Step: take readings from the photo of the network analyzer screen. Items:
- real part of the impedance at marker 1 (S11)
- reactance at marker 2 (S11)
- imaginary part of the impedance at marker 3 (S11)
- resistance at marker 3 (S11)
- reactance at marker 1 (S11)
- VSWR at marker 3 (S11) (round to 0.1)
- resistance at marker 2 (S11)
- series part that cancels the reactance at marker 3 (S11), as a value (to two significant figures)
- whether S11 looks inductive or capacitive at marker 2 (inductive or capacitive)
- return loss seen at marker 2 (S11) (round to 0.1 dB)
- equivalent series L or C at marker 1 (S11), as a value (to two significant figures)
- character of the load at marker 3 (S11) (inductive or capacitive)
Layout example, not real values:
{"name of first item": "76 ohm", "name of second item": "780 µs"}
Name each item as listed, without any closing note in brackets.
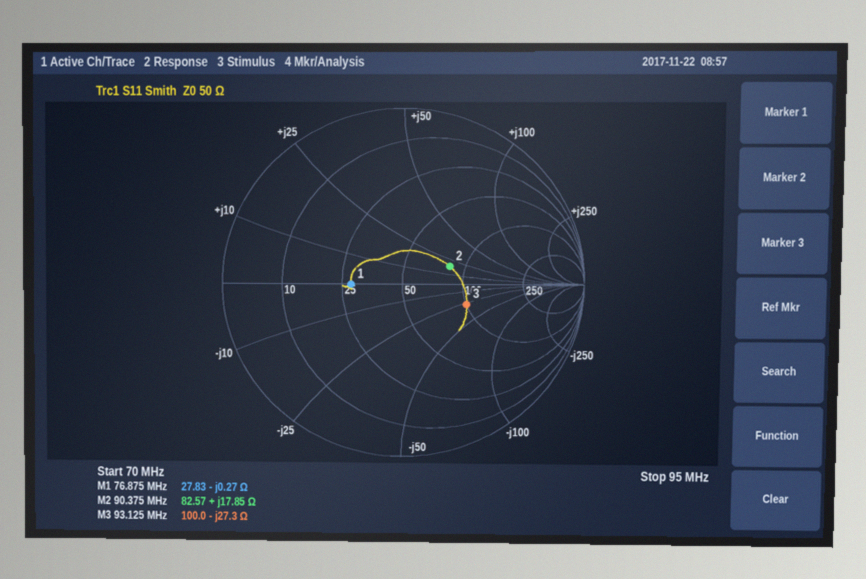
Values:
{"real part of the impedance at marker 1": "27.83 Ω", "reactance at marker 2": "+17.85 Ω", "imaginary part of the impedance at marker 3": "-27.3 Ω", "resistance at marker 3": "100.0 Ω", "reactance at marker 1": "-0.27 Ω", "VSWR at marker 3 (S11)": "2.2", "resistance at marker 2": "82.57 Ω", "series part that cancels the reactance at marker 3 (S11), as a value": "47 nH", "whether S11 looks inductive or capacitive at marker 2": "inductive", "return loss seen at marker 2 (S11)": "11.1 dB", "equivalent series L or C at marker 1 (S11), as a value": "7.7 nF", "character of the load at marker 3 (S11)": "capacitive"}
